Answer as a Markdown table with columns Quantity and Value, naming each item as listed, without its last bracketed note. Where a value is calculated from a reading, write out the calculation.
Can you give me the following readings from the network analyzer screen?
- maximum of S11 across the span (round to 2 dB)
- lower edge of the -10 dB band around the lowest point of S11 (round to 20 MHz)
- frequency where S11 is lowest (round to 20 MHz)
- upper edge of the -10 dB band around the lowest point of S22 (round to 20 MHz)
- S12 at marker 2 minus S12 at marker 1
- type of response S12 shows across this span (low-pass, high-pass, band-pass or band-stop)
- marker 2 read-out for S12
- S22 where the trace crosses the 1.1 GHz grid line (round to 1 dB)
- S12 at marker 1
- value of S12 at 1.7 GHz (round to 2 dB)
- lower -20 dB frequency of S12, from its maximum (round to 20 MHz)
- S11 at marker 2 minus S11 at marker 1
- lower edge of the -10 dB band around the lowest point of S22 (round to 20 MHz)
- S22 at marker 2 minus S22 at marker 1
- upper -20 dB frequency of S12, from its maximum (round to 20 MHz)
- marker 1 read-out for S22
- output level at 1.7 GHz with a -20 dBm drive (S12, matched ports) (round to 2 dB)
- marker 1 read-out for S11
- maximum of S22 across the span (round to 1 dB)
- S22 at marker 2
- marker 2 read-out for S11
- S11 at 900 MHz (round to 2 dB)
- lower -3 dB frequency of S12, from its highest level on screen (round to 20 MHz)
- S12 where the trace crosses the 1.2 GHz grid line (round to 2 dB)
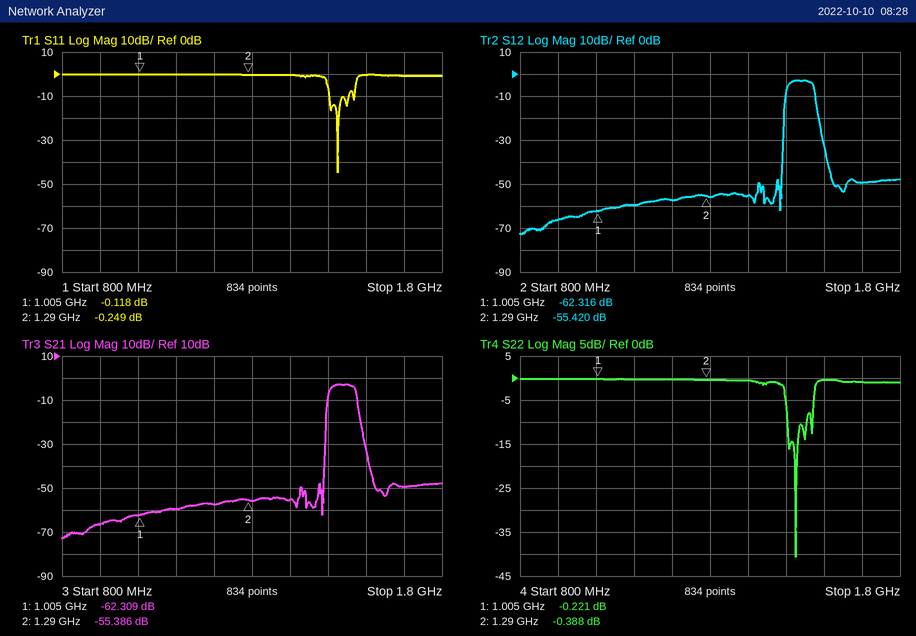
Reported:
| Quantity | Value |
|---|---|
| maximum of S11 across the span | 0 dB |
| lower edge of the -10 dB band around the lowest point of S11 | 1.50 GHz |
| frequency where S11 is lowest | 1.52 GHz |
| upper edge of the -10 dB band around the lowest point of S22 | 1.56 GHz |
| S12 at marker 2 minus S12 at marker 1 | -55.42 − (-62.316) = 6.896 dB |
| type of response S12 shows across this span | band-pass |
| marker 2 read-out for S12 | -55.420 dB |
| S22 where the trace crosses the 1.1 GHz grid line | 0 dB |
| S12 at marker 1 | -62.316 dB |
| value of S12 at 1.7 GHz | -50 dB |
| lower -20 dB frequency of S12, from its maximum | 1.50 GHz |
| S11 at marker 2 minus S11 at marker 1 | -0.249 − (-0.118) = -0.131 dB |
| lower edge of the -10 dB band around the lowest point of S22 | 1.50 GHz |
| S22 at marker 2 minus S22 at marker 1 | -0.388 − (-0.221) = -0.167 dB |
| upper -20 dB frequency of S12, from its maximum | 1.58 GHz |
| marker 1 read-out for S22 | -0.221 dB |
| output level at 1.7 GHz with a -20 dBm drive (S12, matched ports) | -20 dBm + (-50 dB) = -70 dBm |
| marker 1 read-out for S11 | -0.118 dB |
| maximum of S22 across the span | 0 dB |
| S22 at marker 2 | -0.388 dB |
| marker 2 read-out for S11 | -0.249 dB |
| S11 at 900 MHz | 0 dB |
| lower -3 dB frequency of S12, from its highest level on screen | 1.50 GHz |
| S12 where the trace crosses the 1.2 GHz grid line | -58 dB |
